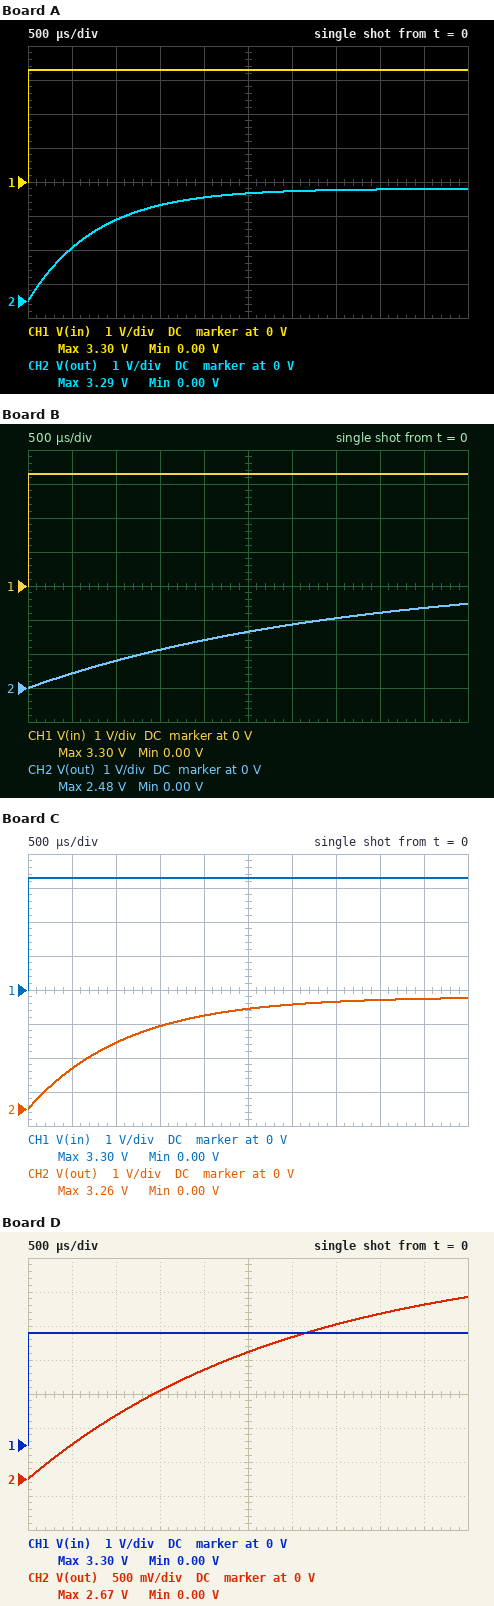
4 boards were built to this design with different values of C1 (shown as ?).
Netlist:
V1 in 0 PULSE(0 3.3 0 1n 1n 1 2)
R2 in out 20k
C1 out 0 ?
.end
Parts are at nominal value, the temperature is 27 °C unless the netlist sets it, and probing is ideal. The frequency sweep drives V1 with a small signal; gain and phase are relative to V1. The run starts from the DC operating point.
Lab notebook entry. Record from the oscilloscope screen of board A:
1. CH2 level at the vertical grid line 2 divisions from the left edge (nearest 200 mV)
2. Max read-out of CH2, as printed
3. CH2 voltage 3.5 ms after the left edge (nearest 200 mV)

2.4 V
3.29 V
3.2 V
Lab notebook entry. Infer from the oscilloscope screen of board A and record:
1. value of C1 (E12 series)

39 nF
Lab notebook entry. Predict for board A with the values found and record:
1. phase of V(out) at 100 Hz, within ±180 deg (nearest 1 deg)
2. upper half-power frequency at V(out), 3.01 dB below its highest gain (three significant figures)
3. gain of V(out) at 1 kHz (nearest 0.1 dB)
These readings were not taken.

-26 deg
204 Hz
-14.0 dB
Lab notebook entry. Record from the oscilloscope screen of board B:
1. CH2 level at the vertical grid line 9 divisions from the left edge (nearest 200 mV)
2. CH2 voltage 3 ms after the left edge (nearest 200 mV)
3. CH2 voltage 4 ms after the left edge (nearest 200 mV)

2.4 V
1.8 V
2.2 V
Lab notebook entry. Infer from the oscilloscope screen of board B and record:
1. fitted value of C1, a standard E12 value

180 nF
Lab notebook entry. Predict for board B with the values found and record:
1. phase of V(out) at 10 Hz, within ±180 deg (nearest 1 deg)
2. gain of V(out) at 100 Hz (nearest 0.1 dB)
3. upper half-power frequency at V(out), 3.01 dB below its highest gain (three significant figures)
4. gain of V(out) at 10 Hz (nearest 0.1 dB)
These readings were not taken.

-13 deg
-7.9 dB
44.2 Hz
-0.2 dB
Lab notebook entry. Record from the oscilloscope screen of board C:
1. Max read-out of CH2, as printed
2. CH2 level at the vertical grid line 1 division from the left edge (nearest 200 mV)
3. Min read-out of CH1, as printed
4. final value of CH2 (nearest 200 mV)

3.26 V
1.2 V
0.00 V
3.2 V
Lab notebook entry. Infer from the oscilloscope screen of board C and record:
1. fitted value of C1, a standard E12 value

56 nF
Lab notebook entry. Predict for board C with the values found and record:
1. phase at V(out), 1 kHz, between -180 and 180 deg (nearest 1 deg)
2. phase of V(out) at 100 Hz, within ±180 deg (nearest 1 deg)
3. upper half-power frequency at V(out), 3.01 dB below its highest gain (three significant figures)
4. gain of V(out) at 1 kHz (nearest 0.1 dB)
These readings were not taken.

-82 deg
-35 deg
142 Hz
-17.0 dB
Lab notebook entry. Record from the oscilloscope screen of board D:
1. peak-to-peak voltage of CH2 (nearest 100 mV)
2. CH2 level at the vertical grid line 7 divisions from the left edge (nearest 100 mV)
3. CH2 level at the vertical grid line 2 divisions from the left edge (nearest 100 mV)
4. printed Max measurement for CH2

2.7 V
2.3 V
900 mV
2.67 V
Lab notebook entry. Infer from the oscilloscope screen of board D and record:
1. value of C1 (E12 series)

150 nF
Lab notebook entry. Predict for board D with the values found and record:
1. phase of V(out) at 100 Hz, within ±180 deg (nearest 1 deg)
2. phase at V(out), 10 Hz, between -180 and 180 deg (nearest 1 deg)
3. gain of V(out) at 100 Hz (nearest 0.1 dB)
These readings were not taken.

-62 deg
-11 deg
-6.6 dB
